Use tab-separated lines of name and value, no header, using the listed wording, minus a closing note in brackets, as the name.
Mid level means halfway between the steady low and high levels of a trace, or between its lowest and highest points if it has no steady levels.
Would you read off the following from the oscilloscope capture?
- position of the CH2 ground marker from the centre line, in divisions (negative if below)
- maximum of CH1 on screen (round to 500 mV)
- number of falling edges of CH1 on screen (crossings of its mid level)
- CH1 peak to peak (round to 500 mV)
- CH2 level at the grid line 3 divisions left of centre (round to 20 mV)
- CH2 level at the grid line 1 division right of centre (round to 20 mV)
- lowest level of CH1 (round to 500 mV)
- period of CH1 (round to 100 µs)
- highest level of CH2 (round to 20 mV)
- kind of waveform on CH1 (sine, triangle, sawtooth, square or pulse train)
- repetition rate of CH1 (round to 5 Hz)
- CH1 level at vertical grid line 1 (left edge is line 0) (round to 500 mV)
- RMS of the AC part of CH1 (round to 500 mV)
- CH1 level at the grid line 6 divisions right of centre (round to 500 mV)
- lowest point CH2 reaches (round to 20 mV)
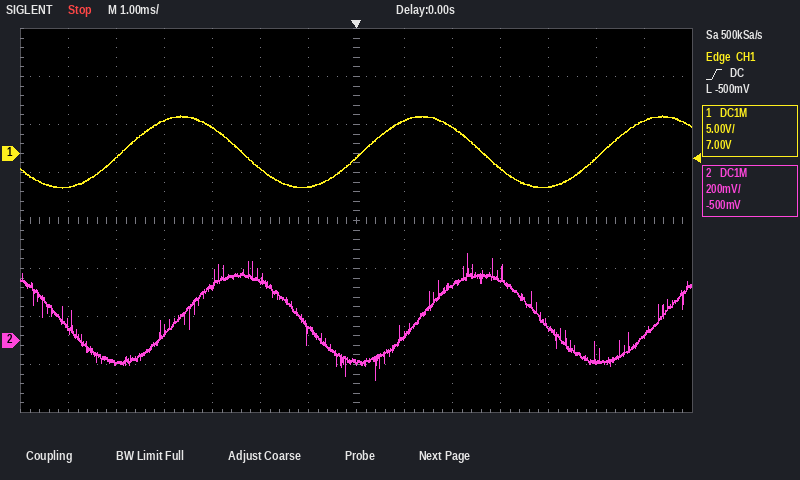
position of the CH2 ground marker from the centre line, in divisions	-2.5 div
maximum of CH1 on screen	4.0 V
number of falling edges of CH1 on screen	2
CH1 peak to peak	7.5 V
CH2 level at the grid line 3 divisions left of centre	220 mV
CH2 level at the grid line 1 division right of centre	20 mV
lowest level of CH1	-3.5 V
period of CH1	5.0 ms
highest level of CH2	360 mV
kind of waveform on CH1	sine
repetition rate of CH1	200 Hz
CH1 level at vertical grid line 1 (left edge is line 0)	-3.5 V
RMS of the AC part of CH1	2.5 V
CH1 level at the grid line 6 divisions right of centre	3.5 V
lowest point CH2 reaches	-160 mV
